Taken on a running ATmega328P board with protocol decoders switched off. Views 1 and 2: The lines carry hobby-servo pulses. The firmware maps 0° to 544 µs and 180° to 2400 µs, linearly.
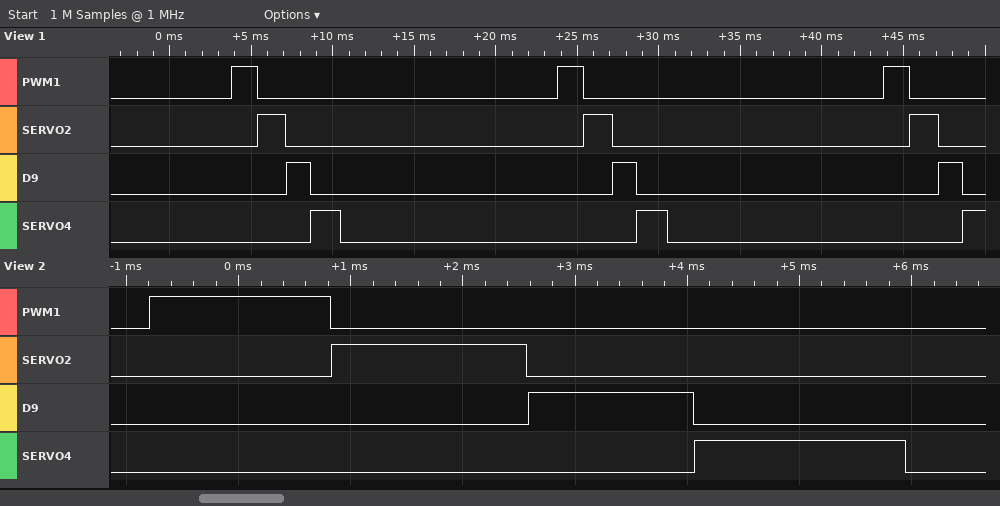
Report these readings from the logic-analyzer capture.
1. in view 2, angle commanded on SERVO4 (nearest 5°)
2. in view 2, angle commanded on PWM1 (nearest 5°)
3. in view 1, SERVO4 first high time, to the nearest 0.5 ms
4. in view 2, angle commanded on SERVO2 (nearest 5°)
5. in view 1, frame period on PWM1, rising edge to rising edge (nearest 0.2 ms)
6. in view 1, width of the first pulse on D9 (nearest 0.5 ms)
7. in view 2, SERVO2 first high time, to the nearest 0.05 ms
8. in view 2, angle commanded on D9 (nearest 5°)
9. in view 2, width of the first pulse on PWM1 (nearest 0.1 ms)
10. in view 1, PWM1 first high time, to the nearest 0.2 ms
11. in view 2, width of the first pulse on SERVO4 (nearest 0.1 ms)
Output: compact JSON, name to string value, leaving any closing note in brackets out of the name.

{"in view 2, angle commanded on SERVO4": "130°", "in view 2, angle commanded on PWM1": "105°", "in view 1, SERVO4 first high time, to the nearest 0.5 ms": "2.0 ms", "in view 2, angle commanded on SERVO2": "115°", "in view 1, frame period on PWM1, rising edge to rising edge": "20.0 ms", "in view 1, width of the first pulse on D9": "1.5 ms", "in view 2, SERVO2 first high time, to the nearest 0.05 ms": "1.75 ms", "in view 2, angle commanded on D9": "90°", "in view 2, width of the first pulse on PWM1": "1.6 ms", "in view 1, PWM1 first high time, to the nearest 0.2 ms": "1.6 ms", "in view 2, width of the first pulse on SERVO4": "1.9 ms"}
